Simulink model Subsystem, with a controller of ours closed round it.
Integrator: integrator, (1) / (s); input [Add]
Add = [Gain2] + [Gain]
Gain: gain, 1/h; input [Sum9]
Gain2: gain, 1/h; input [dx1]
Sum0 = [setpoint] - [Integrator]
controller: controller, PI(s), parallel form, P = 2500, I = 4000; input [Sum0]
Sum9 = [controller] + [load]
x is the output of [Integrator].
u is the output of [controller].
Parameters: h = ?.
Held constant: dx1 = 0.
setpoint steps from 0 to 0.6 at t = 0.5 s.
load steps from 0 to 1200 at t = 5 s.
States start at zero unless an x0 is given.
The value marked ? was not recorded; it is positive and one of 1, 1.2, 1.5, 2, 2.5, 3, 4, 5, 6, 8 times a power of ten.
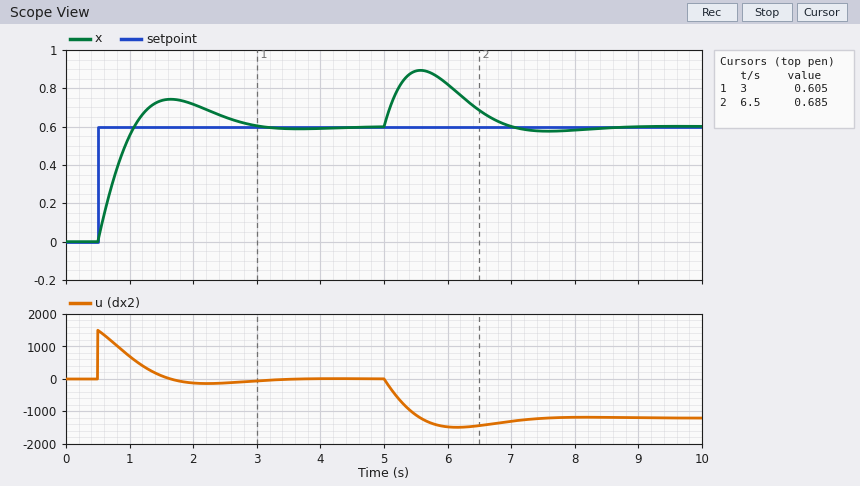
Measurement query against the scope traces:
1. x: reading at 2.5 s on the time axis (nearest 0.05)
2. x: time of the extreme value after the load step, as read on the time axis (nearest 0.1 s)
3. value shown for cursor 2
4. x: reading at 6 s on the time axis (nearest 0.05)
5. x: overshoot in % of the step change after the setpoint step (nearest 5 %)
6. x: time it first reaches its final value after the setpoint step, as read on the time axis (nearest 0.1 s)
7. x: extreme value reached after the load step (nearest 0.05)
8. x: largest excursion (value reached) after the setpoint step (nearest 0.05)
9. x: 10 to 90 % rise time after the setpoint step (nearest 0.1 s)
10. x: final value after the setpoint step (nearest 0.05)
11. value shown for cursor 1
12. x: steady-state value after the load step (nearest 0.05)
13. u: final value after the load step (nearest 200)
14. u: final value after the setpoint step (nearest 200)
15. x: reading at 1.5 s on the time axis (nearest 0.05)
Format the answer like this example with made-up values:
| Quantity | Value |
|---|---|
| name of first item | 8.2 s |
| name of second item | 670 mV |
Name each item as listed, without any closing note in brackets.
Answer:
| Quantity | Value |
|---|---|
| x: reading at 2.5 s on the time axis | 0.65 |
| x: time of the extreme value after the load step, as read on the time axis | 5.6 s |
| value shown for cursor 2 | 0.685 |
| x: reading at 6 s on the time axis | 0.80 |
| x: overshoot in % of the step change after the setpoint step | 25 % |
| x: time it first reaches its final value after the setpoint step, as read on the time axis | 1.1 s |
| x: extreme value reached after the load step | 0.90 |
| x: largest excursion (value reached) after the setpoint step | 0.75 |
| x: 10 to 90 % rise time after the setpoint step | 0.4 s |
| x: final value after the setpoint step | 0.60 |
| value shown for cursor 1 | 0.605 |
| x: steady-state value after the load step | 0.60 |
| u: final value after the load step | -1200 |
| u: final value after the setpoint step | 0 |
| x: reading at 1.5 s on the time axis | 0.75 |
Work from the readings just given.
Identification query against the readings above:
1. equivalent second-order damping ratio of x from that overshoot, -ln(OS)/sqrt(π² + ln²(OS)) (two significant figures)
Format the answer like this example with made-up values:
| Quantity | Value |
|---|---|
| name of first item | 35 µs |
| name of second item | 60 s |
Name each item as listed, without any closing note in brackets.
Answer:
| Quantity | Value |
|---|---|
| equivalent second-order damping ratio of x from that overshoot, -ln(OS)/sqrt(π² + ln²(OS)) | 0.40 |
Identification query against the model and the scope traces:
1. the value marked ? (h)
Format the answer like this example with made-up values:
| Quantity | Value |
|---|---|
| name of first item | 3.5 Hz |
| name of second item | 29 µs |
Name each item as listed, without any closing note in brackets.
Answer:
| Quantity | Value |
|---|---|
| the value marked ? | 1000 |
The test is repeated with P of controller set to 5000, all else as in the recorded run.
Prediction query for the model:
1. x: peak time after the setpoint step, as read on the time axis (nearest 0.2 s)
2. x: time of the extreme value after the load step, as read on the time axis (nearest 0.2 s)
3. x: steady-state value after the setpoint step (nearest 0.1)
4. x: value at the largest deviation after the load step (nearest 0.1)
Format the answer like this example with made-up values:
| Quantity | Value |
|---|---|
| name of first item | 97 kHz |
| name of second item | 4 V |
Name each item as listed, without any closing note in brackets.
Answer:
| Quantity | Value |
|---|---|
| x: peak time after the setpoint step, as read on the time axis | 1.4 s |
| x: time of the extreme value after the load step, as read on the time axis | 5.4 s |
| x: steady-state value after the setpoint step | 0.6 |
| x: value at the largest deviation after the load step | 0.8 |
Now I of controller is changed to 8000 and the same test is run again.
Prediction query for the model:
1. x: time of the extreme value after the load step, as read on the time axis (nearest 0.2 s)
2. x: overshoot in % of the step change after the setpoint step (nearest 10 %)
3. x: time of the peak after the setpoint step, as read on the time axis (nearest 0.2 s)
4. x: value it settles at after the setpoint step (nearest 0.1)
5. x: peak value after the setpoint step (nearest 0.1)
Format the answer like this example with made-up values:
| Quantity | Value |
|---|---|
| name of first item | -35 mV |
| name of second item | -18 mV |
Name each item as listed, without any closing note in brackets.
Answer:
| Quantity | Value |
|---|---|
| x: time of the extreme value after the load step, as read on the time axis | 5.4 s |
| x: overshoot in % of the step change after the setpoint step | 30 % |
| x: time of the peak after the setpoint step, as read on the time axis | 1.4 s |
| x: value it settles at after the setpoint step | 0.6 |
| x: peak value after the setpoint step | 0.8 |
